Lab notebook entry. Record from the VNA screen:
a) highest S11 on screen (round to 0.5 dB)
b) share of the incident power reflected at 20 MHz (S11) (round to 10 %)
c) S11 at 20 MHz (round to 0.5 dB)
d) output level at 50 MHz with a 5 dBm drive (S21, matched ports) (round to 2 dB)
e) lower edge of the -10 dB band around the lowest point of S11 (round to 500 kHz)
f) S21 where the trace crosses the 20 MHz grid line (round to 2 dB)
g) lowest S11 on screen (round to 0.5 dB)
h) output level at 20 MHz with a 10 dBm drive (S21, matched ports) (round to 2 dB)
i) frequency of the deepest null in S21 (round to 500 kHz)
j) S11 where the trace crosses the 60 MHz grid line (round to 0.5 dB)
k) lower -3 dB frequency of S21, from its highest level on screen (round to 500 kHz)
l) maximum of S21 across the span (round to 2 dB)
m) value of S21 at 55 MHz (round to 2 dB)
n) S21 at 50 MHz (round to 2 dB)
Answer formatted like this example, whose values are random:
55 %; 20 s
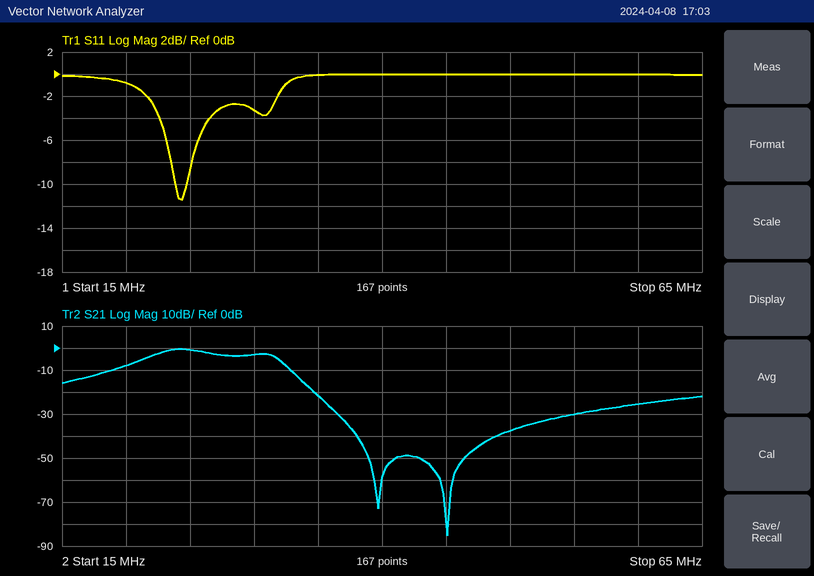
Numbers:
0.0 dB; 80 %; -1.0 dB; -32 dBm; 24.0 MHz; -8 dB; -11.5 dB; 2 dBm; 45.0 MHz; 0.0 dB; 22.0 MHz; 0 dB; -30 dB; -38 dB
